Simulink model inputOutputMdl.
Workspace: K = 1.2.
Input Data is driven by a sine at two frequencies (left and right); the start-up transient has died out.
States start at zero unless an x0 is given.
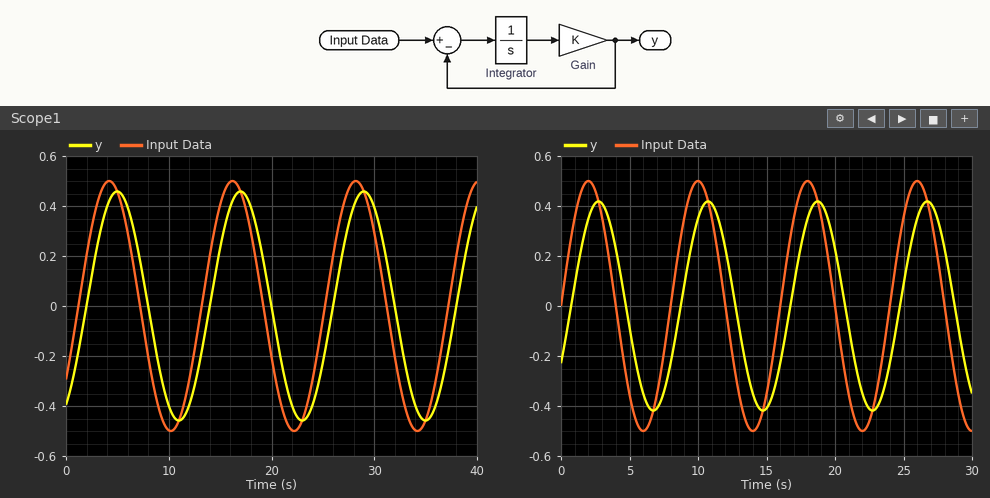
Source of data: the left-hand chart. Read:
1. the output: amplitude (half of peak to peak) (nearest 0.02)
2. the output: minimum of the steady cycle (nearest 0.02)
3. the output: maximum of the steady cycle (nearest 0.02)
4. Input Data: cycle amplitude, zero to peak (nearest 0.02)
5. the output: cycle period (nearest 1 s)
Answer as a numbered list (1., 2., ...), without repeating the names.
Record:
1. 0.46
2. -0.46
3. 0.46
4. 0.50
5. 12 s
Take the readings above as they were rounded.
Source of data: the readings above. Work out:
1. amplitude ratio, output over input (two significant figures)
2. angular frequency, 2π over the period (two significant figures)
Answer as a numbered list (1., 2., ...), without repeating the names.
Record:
1. 0.92
2. 0.52 rad/s
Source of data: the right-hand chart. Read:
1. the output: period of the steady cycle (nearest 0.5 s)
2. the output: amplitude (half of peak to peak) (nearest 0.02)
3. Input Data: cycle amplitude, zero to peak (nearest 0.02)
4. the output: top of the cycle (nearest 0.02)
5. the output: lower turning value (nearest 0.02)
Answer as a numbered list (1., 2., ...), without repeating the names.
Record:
1. 8.0 s
2. 0.42
3. 0.50
4. 0.42
5. -0.42
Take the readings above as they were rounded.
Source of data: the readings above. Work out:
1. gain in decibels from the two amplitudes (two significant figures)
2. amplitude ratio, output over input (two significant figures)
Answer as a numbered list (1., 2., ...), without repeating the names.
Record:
1. -1.5 dB
2. 0.84
